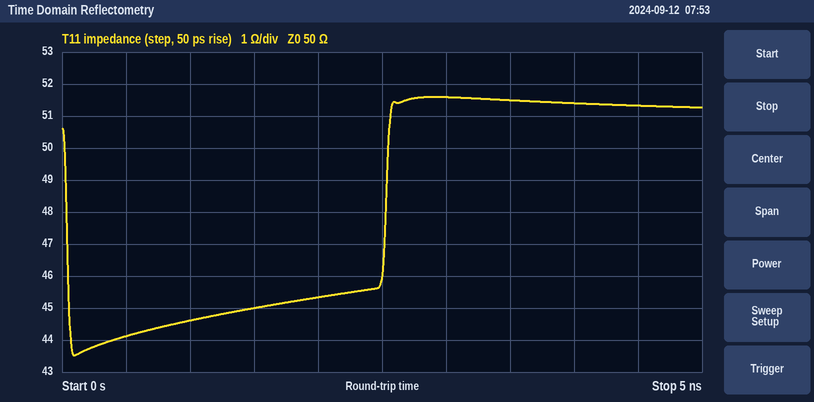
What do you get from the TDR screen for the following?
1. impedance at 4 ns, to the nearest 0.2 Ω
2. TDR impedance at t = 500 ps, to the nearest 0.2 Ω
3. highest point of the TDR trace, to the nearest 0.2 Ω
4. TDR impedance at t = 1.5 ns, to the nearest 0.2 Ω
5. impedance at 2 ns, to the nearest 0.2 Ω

51.4 Ω
44.2 Ω
51.6 Ω
45.0 Ω
45.4 Ω
